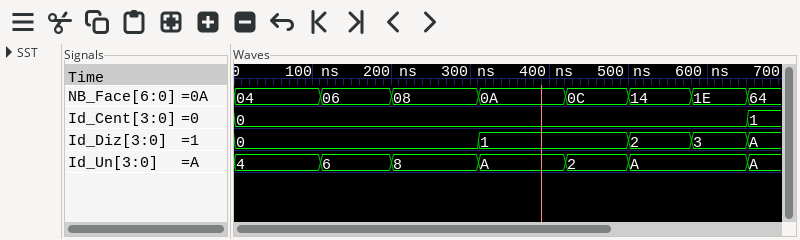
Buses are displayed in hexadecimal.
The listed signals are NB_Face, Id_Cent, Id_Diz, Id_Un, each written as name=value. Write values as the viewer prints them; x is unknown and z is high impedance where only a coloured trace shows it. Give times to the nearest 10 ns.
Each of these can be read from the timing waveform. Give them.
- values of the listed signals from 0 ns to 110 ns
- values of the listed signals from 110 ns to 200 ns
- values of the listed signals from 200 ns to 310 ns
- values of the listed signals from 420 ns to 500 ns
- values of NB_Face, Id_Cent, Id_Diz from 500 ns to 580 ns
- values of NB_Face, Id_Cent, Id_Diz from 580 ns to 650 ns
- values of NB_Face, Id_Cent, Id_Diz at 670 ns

NB_Face=04, Id_Cent=0, Id_Diz=0, Id_Un=4
NB_Face=06, Id_Cent=0, Id_Diz=0, Id_Un=6
NB_Face=08, Id_Cent=0, Id_Diz=0, Id_Un=8
NB_Face=0C, Id_Cent=0, Id_Diz=1, Id_Un=2
NB_Face=14, Id_Cent=0, Id_Diz=2
NB_Face=1E, Id_Cent=0, Id_Diz=3
NB_Face=64, Id_Cent=1, Id_Diz=A
